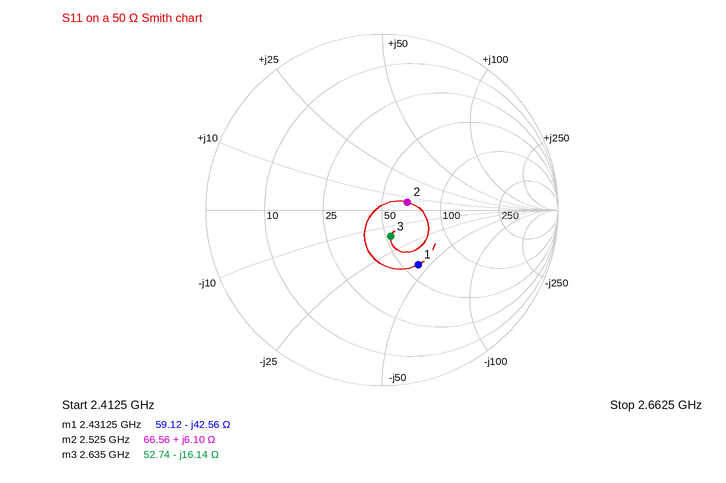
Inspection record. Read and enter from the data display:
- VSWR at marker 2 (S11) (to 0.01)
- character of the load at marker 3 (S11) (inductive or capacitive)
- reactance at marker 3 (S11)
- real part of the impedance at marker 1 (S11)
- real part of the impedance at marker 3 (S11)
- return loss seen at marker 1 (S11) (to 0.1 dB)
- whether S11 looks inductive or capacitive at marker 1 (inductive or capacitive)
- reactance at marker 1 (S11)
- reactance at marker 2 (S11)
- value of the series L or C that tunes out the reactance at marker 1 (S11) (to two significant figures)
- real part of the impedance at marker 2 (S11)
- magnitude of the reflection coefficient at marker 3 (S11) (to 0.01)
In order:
1.36
capacitive
-16.14 Ω
59.12 Ω
52.74 Ω
8.6 dB
capacitive
-42.56 Ω
+6.10 Ω
2.8 nH
66.56 Ω
0.16
